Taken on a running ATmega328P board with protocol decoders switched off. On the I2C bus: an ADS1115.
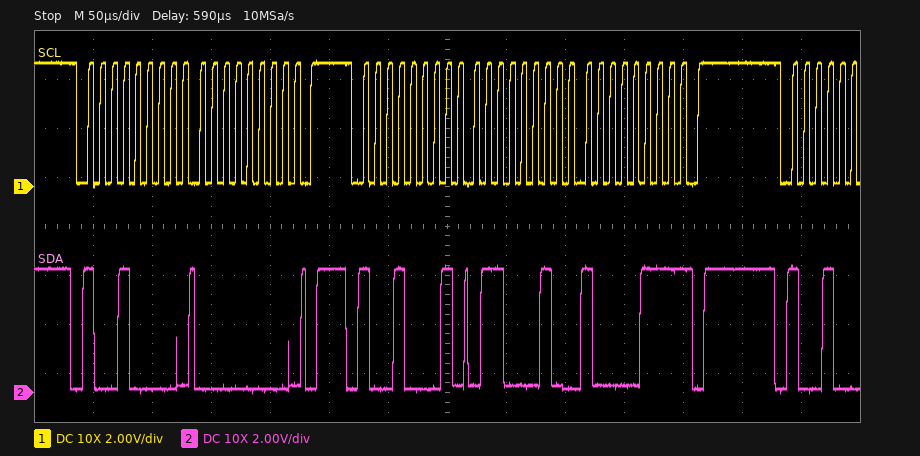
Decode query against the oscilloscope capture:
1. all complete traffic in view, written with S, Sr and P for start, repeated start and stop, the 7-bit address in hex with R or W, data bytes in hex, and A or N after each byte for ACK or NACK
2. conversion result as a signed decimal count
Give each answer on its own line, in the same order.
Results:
S 48W A 00 A P S 48R A 62 A 87 N P
25223
